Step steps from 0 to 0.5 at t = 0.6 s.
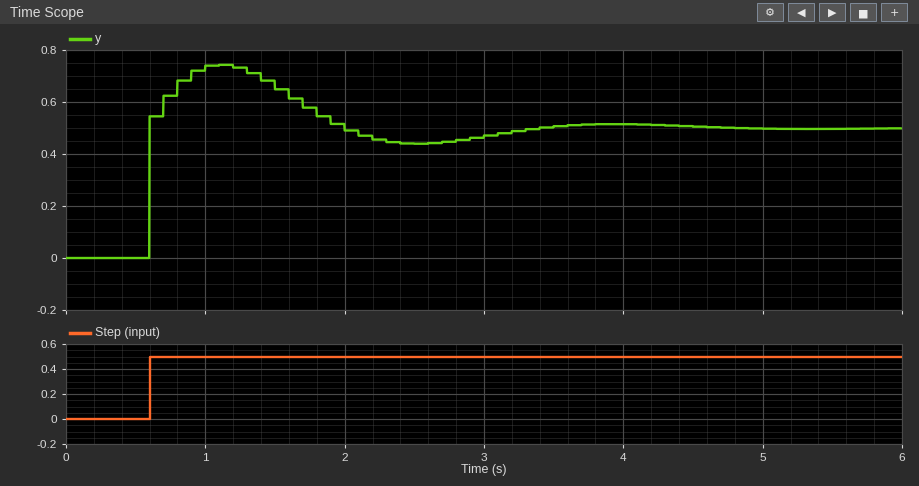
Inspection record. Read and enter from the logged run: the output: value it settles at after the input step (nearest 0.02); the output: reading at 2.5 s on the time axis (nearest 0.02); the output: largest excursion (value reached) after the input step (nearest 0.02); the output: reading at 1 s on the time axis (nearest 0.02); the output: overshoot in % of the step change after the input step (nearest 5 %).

0.50
0.44
0.74
0.74
50 %
